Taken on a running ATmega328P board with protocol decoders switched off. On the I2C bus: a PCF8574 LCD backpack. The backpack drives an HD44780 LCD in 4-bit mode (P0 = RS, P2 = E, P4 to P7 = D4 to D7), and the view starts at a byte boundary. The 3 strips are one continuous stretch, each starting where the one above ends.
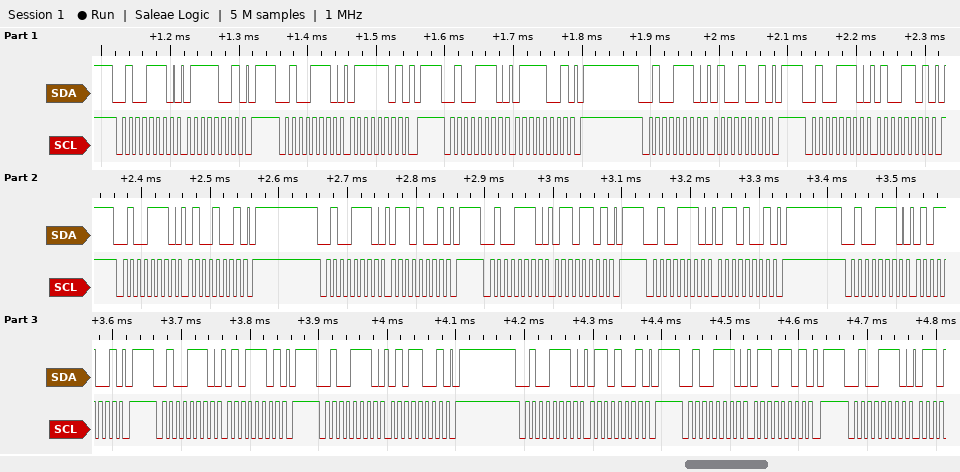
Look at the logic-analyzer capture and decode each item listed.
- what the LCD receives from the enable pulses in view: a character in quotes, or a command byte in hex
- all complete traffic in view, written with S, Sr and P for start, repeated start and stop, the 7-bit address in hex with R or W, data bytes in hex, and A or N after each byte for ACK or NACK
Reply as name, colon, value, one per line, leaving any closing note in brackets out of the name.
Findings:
what the LCD receives from the enable pulses in view: a character in quotes, or a command byte in hex: 't' 'e'
all complete traffic in view, written with S, Sr and P for start, repeated start and stop, the 7-bit address in hex with R or W, data bytes in hex, and A or N after each byte for ACK or NACK: S 27W A 79 A P S 27W A 7D A P S 27W A 79 A P S 27W A 49 A P S 27W A 4D A P S 27W A 49 A P S 27W A 69 A P S 27W A 6D A P S 27W A 69 A P S 27W A 59 A P S 27W A 5D A P S 27W A 59 A P S 27W A 69 A P S 27W A 6D A P S 27W A
